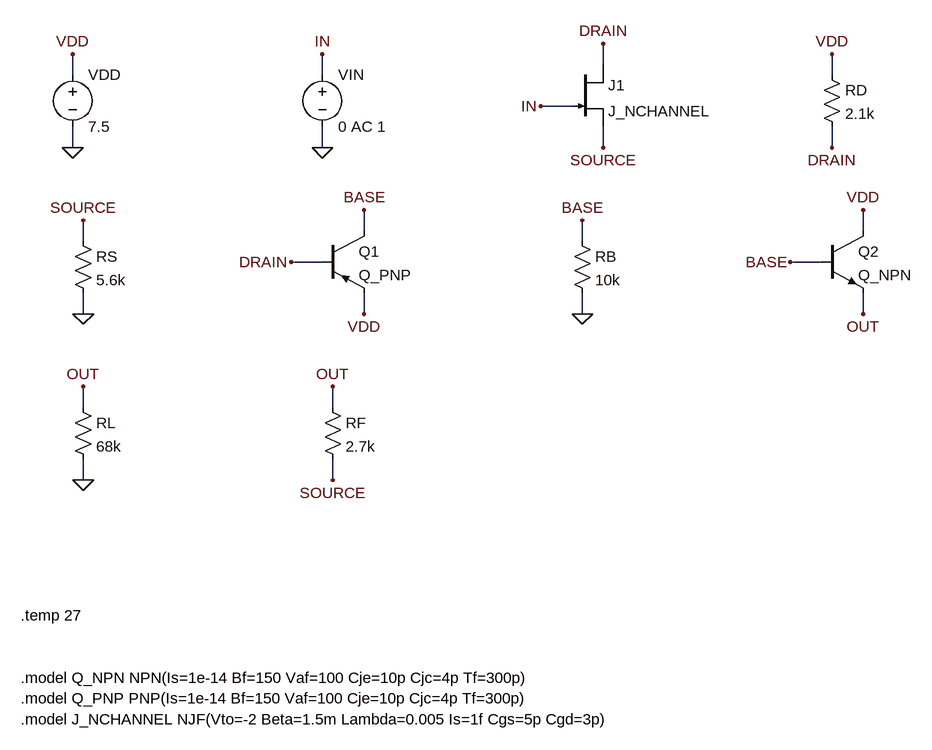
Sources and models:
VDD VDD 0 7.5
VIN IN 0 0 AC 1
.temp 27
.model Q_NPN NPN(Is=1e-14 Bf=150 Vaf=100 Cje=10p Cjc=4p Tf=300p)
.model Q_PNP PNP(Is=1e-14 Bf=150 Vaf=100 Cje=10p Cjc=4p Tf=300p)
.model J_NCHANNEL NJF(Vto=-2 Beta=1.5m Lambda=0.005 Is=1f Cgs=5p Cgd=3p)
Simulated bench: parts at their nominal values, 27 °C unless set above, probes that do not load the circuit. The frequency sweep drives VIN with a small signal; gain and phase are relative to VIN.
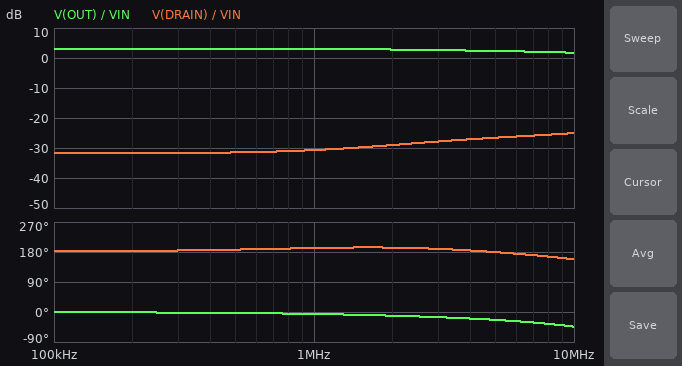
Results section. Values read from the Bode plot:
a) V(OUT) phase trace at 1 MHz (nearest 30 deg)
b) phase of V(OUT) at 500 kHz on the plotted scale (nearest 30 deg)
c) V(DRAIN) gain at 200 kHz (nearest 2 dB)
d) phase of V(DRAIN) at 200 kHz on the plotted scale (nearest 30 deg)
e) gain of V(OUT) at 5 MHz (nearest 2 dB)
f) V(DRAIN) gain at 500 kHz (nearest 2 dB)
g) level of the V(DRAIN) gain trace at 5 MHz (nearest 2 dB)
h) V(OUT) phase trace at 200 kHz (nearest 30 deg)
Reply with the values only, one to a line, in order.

0 deg
0 deg
-32 dB
180 deg
2 dB
-32 dB
-26 dB
0 deg
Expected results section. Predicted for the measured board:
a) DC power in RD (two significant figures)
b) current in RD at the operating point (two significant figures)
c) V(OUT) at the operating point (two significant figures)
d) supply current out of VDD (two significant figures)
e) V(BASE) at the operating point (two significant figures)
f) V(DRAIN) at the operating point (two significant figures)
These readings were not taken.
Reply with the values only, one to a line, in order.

180 µW
290 µA
1.5 V
510 µA
2.1 V
6.9 V
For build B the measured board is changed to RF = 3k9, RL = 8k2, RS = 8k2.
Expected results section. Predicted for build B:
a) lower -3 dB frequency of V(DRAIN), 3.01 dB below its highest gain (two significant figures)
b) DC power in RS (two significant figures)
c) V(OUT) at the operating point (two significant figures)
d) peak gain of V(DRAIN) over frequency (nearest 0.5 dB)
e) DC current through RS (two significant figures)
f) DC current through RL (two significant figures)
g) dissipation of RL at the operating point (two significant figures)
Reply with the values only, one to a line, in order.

7.1 MHz
300 µW
1.2 V
-21.0 dB
190 µA
140 µA
170 µW
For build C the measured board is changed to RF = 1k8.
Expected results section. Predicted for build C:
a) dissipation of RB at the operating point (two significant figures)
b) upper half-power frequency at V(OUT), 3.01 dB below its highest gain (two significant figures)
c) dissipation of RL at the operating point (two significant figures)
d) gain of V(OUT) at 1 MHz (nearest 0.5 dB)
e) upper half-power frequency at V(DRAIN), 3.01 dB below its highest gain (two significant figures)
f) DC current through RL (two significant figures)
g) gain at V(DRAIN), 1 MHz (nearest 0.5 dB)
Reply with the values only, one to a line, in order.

430 µW
23 MHz
35 µW
2.0 dB
260 MHz
23 µA
-31.5 dB
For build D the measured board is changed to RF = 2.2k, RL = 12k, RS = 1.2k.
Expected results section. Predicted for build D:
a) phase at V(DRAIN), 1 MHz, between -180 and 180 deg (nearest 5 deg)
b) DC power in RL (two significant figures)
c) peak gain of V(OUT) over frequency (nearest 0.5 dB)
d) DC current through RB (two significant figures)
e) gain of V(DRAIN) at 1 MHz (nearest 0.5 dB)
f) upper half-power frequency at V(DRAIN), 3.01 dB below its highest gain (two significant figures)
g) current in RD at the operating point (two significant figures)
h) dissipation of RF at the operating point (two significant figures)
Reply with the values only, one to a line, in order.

-170 deg
1.2 mW
9.0 dB
440 µA
-35.0 dB
170 MHz
300 µA
2.2 mW
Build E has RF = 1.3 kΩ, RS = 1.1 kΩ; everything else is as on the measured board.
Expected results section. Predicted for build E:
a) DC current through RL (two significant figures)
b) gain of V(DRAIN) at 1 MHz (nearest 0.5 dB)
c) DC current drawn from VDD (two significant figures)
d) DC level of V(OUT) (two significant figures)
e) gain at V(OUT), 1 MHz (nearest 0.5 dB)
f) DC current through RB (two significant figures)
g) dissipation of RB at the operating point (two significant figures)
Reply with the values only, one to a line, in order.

44 µA
-35.5 dB
1.8 mA
3.0 V
6.5 dB
370 µA
1.3 mW
